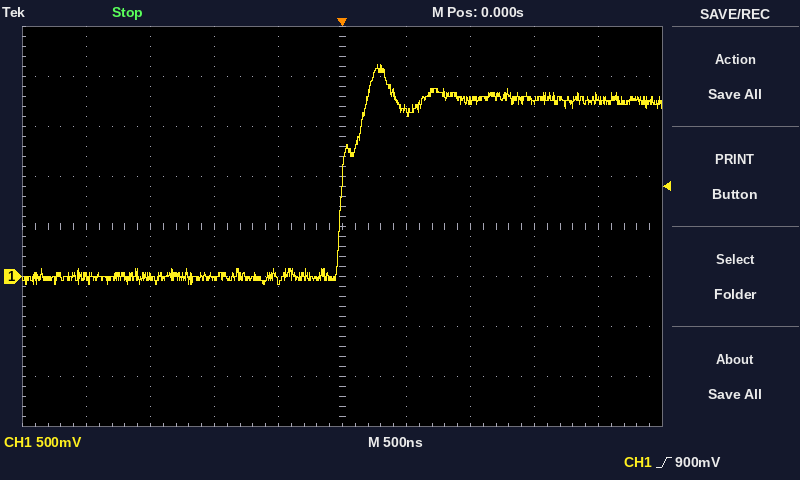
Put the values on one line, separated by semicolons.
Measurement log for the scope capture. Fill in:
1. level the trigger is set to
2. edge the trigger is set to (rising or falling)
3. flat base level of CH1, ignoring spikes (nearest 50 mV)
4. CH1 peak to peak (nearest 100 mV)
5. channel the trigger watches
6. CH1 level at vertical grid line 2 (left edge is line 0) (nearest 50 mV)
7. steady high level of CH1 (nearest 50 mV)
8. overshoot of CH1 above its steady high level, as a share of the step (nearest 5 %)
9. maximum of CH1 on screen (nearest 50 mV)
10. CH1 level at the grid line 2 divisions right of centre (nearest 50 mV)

900 mV; rising; 0 mV; 2.20 V; CH1; 0 mV; 1.75 V; 20 %; 2.10 V; 1.75 V
